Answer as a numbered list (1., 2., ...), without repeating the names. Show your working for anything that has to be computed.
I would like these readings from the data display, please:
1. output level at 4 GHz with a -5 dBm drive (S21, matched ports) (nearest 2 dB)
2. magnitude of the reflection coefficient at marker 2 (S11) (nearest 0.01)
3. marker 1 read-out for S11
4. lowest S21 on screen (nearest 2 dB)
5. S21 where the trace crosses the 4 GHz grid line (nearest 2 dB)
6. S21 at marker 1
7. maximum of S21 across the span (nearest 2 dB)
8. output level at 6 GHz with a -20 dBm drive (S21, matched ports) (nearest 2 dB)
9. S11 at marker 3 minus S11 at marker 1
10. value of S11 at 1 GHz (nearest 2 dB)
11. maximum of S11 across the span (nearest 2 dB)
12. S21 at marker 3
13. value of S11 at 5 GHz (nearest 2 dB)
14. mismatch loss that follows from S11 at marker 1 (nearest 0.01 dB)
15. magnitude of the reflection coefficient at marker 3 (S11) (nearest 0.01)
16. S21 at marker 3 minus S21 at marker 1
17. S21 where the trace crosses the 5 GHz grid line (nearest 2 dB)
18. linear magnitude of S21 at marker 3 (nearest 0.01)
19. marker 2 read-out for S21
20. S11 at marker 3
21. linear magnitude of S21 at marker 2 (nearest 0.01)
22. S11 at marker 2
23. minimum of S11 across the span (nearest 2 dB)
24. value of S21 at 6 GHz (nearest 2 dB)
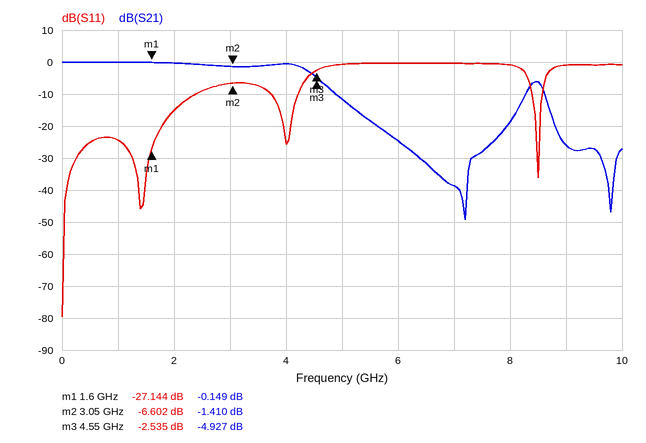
1. -5 dBm + (0 dB) = -6 dBm
2. 10^(-6.602/20) ≈ 0.47
3. -27.144 dB
4. -50 dB
5. 0 dB
6. -0.149 dB
7. 0 dB
8. -20 dBm + (-24 dB) = -44 dBm
9. -2.535 − (-27.144) = 24.609 dB
10. -24 dB
11. 0 dB
12. -4.927 dB
13. 0 dB
14. −10 log10(1 − 10^(-27.144/10)) ≈ 0.01 dB
15. 10^(-2.535/20) ≈ 0.75
16. -4.927 − (-0.149) = -4.778 dB
17. -12 dB
18. 10^(-4.927/20) ≈ 0.57
19. -1.410 dB
20. -2.535 dB
21. 10^(-1.41/20) ≈ 0.85
22. -6.602 dB
23. -80 dB
24. -24 dB
